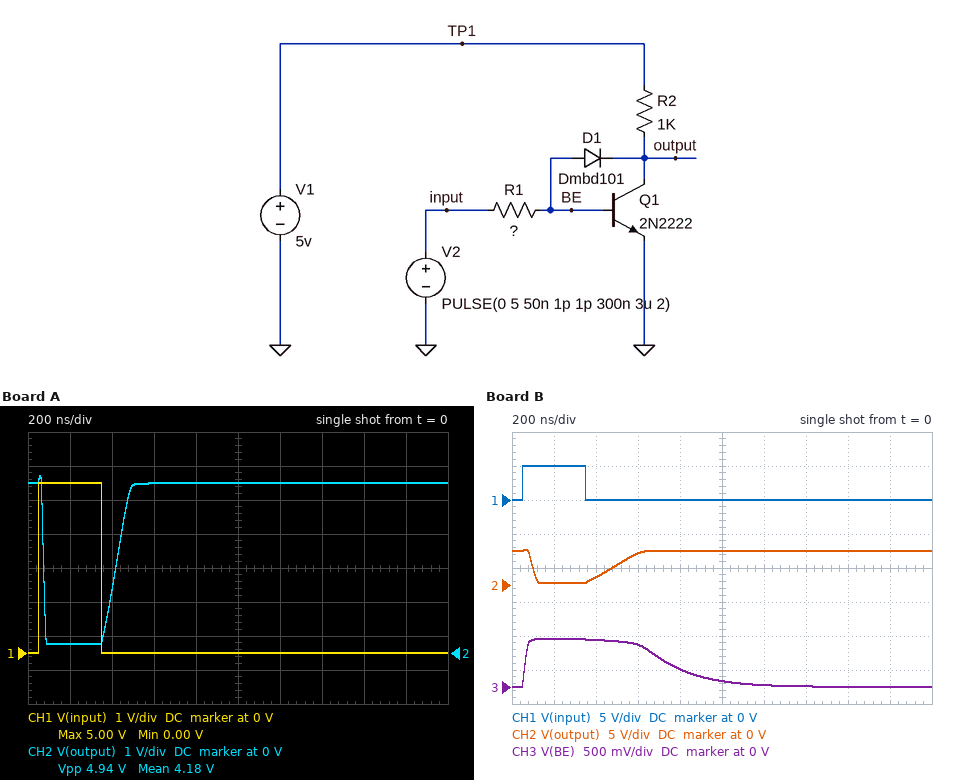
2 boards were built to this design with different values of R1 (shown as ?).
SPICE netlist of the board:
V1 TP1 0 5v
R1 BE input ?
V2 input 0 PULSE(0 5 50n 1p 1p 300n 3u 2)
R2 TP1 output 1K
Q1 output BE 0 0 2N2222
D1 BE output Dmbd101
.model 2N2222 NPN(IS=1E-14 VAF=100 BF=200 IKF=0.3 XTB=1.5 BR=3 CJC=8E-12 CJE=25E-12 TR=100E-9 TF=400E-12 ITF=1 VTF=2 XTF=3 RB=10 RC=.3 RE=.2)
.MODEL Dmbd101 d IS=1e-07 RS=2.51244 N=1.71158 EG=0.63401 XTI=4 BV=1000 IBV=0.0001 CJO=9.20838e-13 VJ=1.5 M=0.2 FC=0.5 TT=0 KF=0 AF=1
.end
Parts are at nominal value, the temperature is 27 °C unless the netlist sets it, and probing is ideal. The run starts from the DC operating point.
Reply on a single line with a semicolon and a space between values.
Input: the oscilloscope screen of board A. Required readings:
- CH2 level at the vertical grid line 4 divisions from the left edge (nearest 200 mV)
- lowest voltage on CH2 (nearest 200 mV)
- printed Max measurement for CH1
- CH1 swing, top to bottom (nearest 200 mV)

5.0 V; 200 mV; 5.00 V; 5.0 V
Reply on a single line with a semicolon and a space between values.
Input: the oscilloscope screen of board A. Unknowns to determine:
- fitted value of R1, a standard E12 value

2.7 kΩ
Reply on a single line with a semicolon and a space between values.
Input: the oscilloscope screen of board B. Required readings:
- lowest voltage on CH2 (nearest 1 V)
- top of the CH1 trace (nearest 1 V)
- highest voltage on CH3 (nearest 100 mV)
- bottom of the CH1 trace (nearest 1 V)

0 V; 5 V; 700 mV; 0 V
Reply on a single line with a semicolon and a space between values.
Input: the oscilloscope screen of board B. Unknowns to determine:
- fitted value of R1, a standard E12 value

5.6 kΩ
